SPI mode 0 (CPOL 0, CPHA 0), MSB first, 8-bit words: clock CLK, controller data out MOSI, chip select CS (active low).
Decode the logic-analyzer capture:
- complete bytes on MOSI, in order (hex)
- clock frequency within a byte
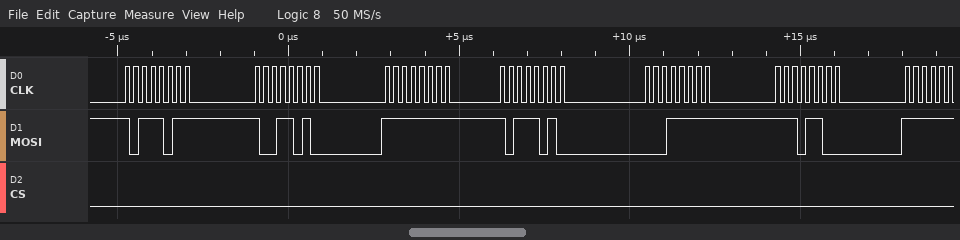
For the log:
0xBB 0x9A 0xFF 0xBA 0x1F 0xEC
4 MHz
